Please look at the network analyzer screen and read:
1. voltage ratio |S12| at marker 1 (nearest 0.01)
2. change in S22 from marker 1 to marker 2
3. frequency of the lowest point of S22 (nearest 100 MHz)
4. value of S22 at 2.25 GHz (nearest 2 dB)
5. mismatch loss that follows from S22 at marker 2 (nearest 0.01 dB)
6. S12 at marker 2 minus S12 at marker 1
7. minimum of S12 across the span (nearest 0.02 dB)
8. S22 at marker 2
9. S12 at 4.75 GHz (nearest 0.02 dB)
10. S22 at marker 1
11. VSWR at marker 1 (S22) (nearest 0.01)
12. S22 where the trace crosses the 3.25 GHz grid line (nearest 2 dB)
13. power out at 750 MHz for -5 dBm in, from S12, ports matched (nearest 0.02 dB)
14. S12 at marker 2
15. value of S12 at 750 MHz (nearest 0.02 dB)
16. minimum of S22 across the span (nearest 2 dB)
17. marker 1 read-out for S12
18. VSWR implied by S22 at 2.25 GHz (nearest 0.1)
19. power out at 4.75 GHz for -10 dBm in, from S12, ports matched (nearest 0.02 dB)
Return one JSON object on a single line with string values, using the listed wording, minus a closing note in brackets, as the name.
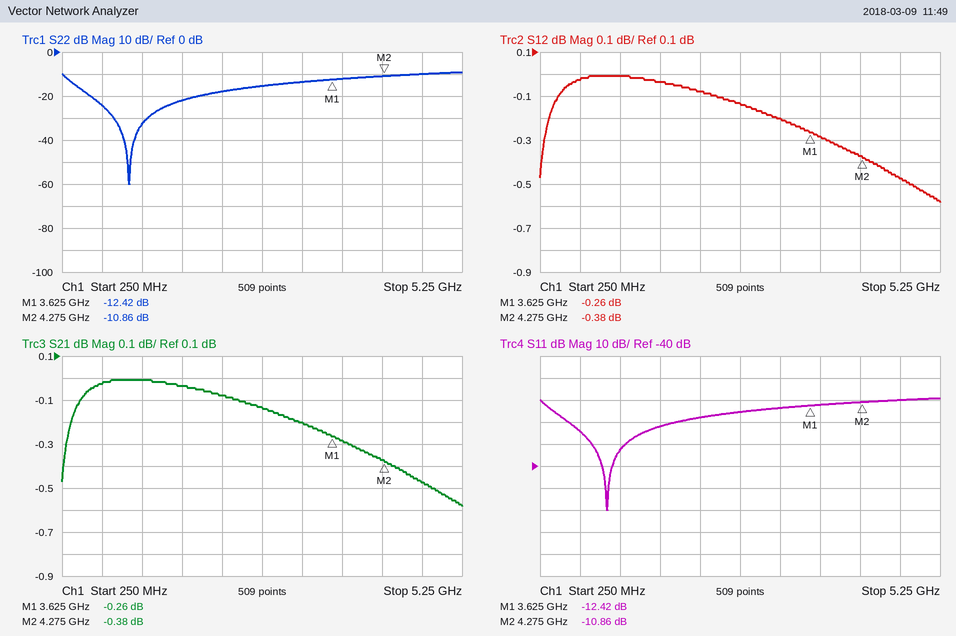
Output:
{"voltage ratio |S12| at marker 1": "0.97", "change in S22 from marker 1 to marker 2": "1.56 dB", "frequency of the lowest point of S22": "1.1 GHz", "value of S22 at 2.25 GHz": "-18 dB", "mismatch loss that follows from S22 at marker 2": "0.37 dB", "S12 at marker 2 minus S12 at marker 1": "-0.12 dB", "minimum of S12 across the span": "-0.58 dB", "S22 at marker 2": "-10.86 dB", "S12 at 4.75 GHz": "-0.48 dB", "S22 at marker 1": "-12.42 dB", "VSWR at marker 1 (S22)": "1.63", "S22 where the trace crosses the 3.25 GHz grid line": "-14 dB", "power out at 750 MHz for -5 dBm in, from S12, ports matched": "-5.02 dBm", "S12 at marker 2": "-0.38 dB", "value of S12 at 750 MHz": "-0.02 dB", "minimum of S22 across the span": "-60 dB", "marker 1 read-out for S12": "-0.26 dB", "VSWR implied by S22 at 2.25 GHz": "1.3", "power out at 4.75 GHz for -10 dBm in, from S12, ports matched": "-10.48 dBm"}
